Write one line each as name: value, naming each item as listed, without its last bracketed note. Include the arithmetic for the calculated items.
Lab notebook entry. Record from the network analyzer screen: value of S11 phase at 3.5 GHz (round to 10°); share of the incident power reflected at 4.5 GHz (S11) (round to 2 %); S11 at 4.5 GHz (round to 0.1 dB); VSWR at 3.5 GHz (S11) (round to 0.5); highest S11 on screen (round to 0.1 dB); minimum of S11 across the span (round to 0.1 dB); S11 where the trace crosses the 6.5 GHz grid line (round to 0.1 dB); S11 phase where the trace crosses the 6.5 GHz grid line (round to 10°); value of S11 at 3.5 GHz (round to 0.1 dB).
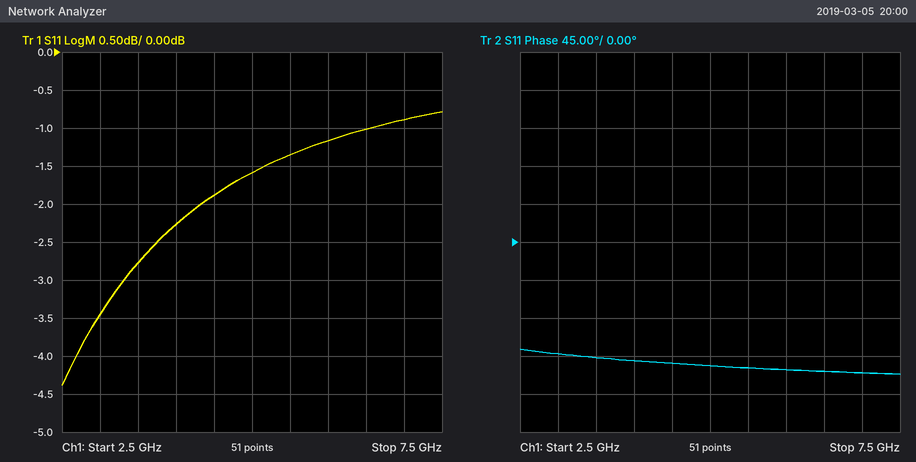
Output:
value of S11 phase at 3.5 GHz: -140°
share of the incident power reflected at 4.5 GHz (S11): 10^(-1.9/10) ≈ 64.6 %, so 64 % to the nearest 2 %
S11 at 4.5 GHz: -1.9 dB
VSWR at 3.5 GHz (S11): |Γ| = 10^(-2.8/20) = 0.7244; VSWR = (1 + 0.7244)/(1 − 0.7244) ≈ 6.26, so 6.5 to the nearest 0.5
highest S11 on screen: -0.8 dB
minimum of S11 across the span: -4.4 dB
S11 where the trace crosses the 6.5 GHz grid line: -1.0 dB
S11 phase where the trace crosses the 6.5 GHz grid line: -150°
value of S11 at 3.5 GHz: -2.8 dB
